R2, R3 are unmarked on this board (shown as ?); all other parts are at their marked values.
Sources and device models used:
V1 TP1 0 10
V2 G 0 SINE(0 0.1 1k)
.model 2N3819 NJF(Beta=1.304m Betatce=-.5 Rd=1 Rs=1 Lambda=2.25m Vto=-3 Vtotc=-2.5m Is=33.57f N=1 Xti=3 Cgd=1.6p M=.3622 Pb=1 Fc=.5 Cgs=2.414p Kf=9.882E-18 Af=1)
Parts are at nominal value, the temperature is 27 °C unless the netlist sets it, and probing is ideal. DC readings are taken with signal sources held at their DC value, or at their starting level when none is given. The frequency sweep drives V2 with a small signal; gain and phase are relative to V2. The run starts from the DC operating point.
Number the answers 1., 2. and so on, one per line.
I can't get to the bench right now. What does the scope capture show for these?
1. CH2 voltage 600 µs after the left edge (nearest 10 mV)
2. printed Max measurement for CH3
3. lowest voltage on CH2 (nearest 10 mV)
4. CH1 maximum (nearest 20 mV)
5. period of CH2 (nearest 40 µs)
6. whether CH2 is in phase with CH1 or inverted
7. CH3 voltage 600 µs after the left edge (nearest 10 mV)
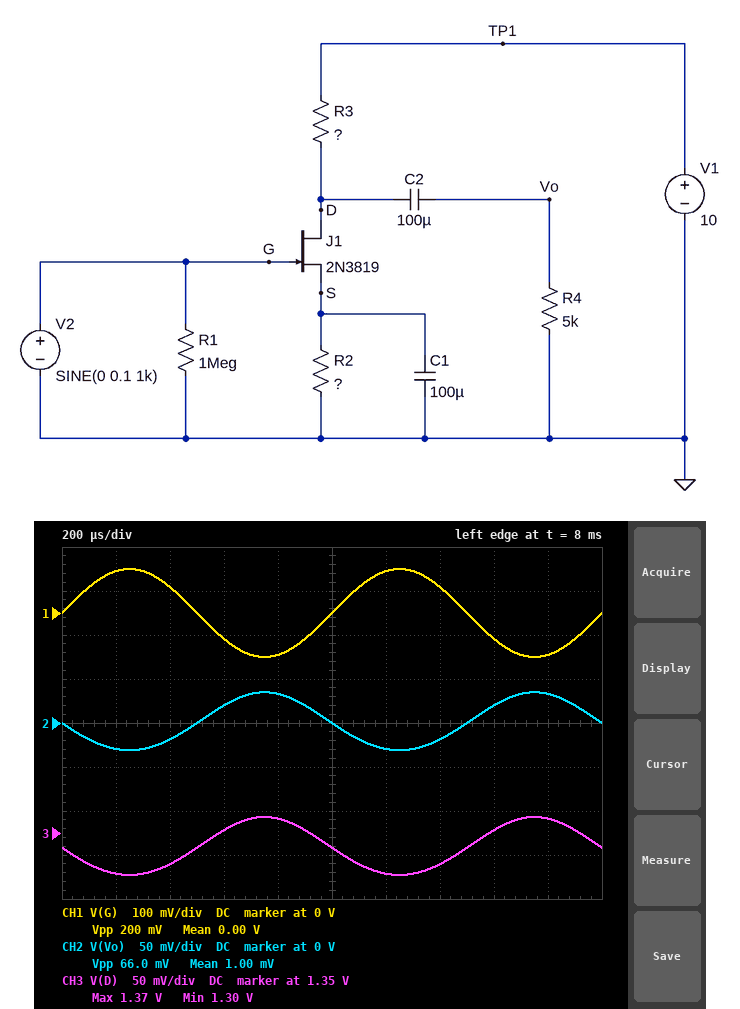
1. 20 mV
2. 1.37 V
3. -30 mV
4. 100 mV
5. 1.00 ms
6. inverted
7. 1.35 V
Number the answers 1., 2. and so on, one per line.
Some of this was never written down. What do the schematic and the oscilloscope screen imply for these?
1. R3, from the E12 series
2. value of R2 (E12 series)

1. 2.7 kΩ
2. 220 Ω
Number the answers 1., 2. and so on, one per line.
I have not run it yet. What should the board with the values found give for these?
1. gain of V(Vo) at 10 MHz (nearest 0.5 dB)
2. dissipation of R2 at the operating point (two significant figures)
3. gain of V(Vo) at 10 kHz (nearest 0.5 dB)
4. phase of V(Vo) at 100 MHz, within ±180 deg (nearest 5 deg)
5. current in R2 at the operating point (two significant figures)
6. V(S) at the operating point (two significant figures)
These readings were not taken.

1. -9.5 dB
2. 2.3 mW
3. -9.5 dB
4. 150 deg
5. 3.2 mA
6. 710 mV
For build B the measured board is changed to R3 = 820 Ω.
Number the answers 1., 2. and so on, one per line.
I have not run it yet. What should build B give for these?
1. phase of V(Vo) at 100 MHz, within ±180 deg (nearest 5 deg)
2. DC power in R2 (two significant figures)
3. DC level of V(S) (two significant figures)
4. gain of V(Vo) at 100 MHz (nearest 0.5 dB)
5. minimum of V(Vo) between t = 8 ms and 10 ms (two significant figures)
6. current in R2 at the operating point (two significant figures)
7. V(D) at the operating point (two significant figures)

1. 160 deg
2. 5.2 mW
3. 1.1 V
4. 10.5 dB
5. -360 mV
6. 4.9 mA
7. 6.0 V
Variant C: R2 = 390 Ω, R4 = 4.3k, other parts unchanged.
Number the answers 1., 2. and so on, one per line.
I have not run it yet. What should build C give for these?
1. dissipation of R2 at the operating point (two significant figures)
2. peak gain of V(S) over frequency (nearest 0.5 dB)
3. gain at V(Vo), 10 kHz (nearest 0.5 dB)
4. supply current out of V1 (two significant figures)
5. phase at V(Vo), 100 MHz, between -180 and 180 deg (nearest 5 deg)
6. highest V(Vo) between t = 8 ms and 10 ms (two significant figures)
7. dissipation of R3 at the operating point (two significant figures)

1. 3.5 mW
2. -19.5 dB
3. -4.0 dB
4. 3.0 mA
5. 155 deg
6. 69 mV
7. 24 mW
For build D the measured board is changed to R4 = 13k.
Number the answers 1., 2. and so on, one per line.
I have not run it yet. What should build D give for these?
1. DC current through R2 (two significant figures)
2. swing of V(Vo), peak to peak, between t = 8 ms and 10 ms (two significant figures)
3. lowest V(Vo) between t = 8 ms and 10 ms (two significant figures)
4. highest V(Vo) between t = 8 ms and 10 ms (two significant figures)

1. 3.2 mA
2. 68 mV
3. -32 mV
4. 36 mV
